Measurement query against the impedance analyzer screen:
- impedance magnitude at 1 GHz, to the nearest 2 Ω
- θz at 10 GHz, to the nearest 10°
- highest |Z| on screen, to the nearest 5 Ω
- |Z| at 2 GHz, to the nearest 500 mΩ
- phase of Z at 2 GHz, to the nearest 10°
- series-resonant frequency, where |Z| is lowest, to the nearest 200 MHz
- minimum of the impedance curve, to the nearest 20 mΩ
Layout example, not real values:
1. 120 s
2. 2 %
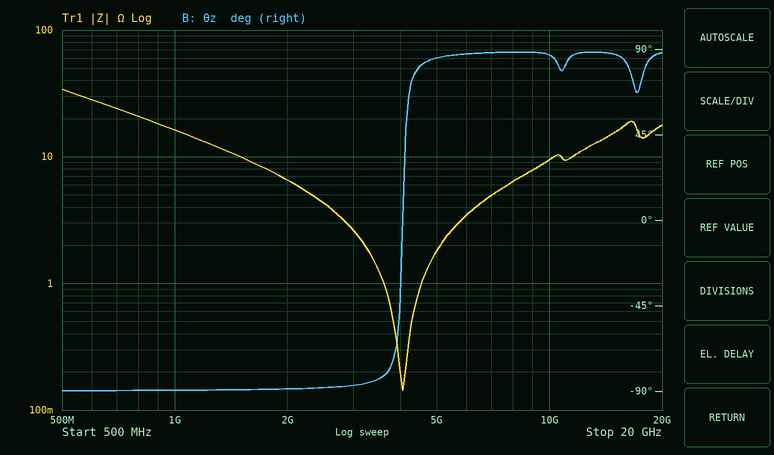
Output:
1. 16 Ω
2. 90°
3. 35 Ω
4. 6.5 Ω
5. -90°
6. 4.0 GHz
7. 140 mΩ
